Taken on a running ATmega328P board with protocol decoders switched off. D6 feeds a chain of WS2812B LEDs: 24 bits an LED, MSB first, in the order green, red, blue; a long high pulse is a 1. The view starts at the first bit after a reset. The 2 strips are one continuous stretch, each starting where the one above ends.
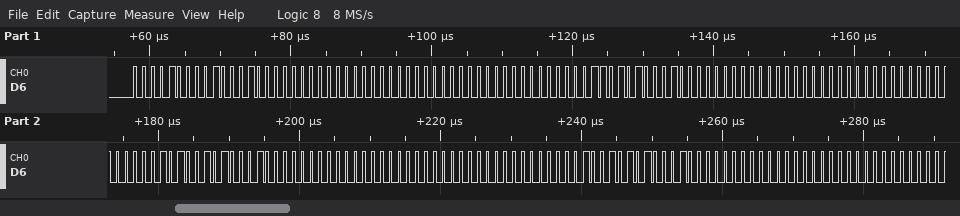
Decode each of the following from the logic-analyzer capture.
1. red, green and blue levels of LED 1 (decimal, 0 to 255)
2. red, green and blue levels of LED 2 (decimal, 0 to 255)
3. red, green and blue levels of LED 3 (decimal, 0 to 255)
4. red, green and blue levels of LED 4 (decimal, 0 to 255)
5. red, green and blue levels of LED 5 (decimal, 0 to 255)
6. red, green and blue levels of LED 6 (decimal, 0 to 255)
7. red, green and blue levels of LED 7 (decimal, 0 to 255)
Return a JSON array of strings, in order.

["68, 8, 0", "0, 0, 0", "68, 13, 0", "0, 0, 0", "68, 41, 0", "0, 0, 0", "68, 37, 0"]
